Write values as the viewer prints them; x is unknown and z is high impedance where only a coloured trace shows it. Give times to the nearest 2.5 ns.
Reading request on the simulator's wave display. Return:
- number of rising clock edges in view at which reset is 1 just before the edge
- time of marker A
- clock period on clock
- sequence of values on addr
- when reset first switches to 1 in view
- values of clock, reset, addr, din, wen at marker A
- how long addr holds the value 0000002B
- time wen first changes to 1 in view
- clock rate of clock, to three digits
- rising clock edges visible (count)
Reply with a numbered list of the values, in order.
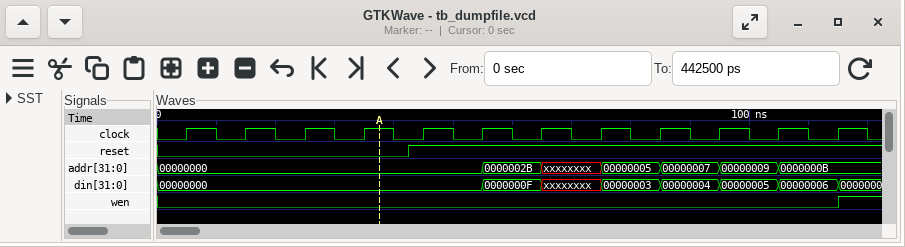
1. 8
2. 37.5 ns
3. 10 ns
4. 00000000, 0000002B, xxxxxxxx, 00000005, 00000007, 00000009, 0000000B
5. 42.5 ns
6. clock=1, reset=0, addr=00000000, din=00000000, wen=0
7. 10 ns
8. 115 ns
9. 100 MHz
10. 12
